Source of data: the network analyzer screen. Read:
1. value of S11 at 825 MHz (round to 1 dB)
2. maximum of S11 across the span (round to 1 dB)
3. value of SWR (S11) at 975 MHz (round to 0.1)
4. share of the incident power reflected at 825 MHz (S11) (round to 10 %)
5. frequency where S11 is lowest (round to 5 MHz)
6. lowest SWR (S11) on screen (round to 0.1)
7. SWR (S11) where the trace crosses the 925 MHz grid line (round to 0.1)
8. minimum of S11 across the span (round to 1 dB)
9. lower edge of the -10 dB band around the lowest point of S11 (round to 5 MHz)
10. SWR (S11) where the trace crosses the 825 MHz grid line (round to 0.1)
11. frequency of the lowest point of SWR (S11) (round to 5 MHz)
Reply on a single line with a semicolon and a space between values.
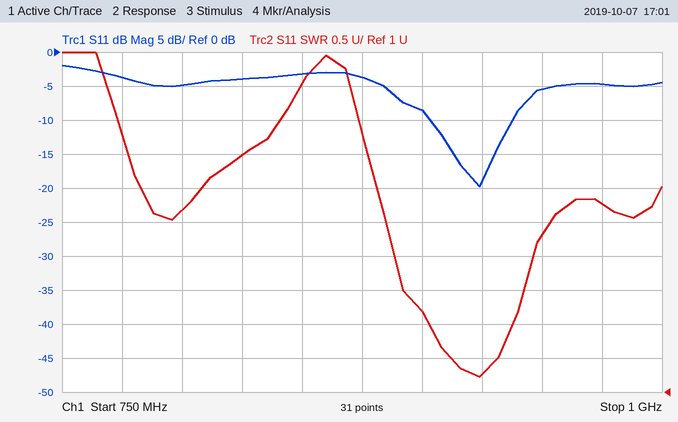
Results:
-4 dB; -2 dB; 3.8; 40 %; 925 MHz; 1.2; 1.3; -20 dB; 905 MHz; 4.5; 925 MHz
